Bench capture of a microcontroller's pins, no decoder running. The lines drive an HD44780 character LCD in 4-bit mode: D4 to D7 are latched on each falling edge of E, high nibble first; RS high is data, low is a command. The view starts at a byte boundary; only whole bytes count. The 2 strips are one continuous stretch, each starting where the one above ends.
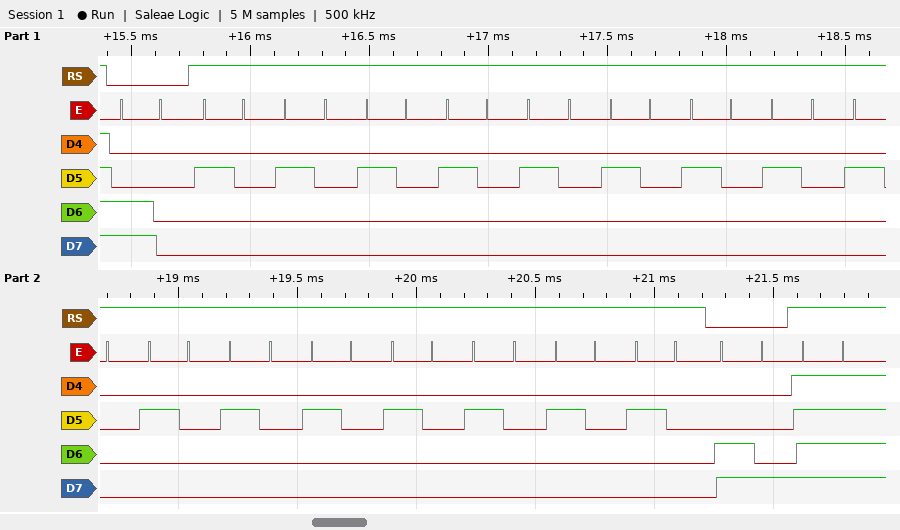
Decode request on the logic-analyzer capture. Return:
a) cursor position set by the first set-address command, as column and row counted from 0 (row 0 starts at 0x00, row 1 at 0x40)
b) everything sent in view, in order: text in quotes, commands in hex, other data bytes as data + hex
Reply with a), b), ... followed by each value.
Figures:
a) column 0, row 1
b) 0xC0 "                " 0xC8 data FF
